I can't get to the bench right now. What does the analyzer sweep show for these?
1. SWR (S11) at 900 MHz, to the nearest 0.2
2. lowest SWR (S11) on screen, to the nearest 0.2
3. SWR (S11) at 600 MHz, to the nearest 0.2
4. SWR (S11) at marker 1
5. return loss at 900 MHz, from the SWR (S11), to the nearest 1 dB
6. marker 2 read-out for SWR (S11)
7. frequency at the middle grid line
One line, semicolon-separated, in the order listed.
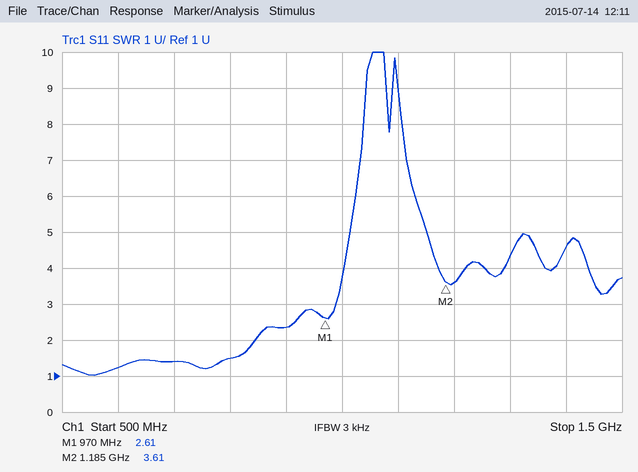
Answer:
2.4; 1.0; 1.2; 2.61; 8 dB; 3.61; 1 GHz
